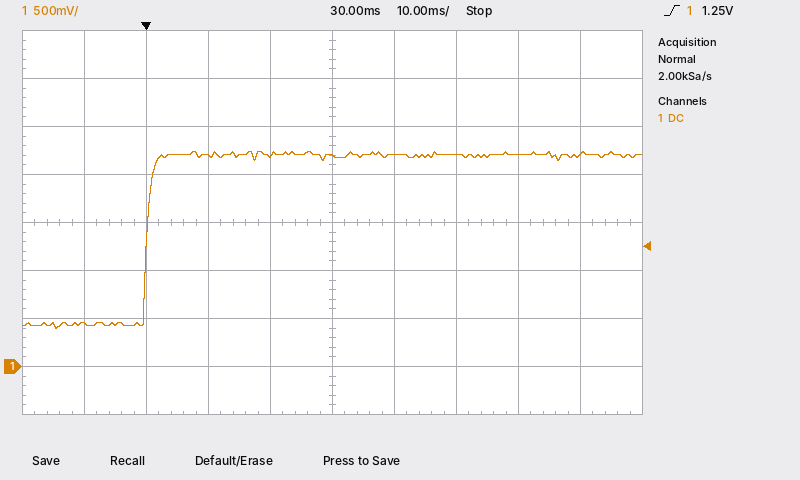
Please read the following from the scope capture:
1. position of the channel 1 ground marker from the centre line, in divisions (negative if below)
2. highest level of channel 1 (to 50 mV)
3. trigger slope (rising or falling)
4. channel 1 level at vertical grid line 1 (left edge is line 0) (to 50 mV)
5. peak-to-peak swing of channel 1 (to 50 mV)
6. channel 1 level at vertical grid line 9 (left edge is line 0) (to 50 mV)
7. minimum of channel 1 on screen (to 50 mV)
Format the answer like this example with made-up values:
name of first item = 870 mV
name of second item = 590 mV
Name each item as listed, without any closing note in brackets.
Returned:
position of the channel 1 ground marker from the centre line, in divisions = -3.0 div
highest level of channel 1 = 2.25 V
trigger slope = rising
channel 1 level at vertical grid line 1 (left edge is line 0) = 450 mV
peak-to-peak swing of channel 1 = 1.85 V
channel 1 level at vertical grid line 9 (left edge is line 0) = 2.20 V
minimum of channel 1 on screen = 400 mV
